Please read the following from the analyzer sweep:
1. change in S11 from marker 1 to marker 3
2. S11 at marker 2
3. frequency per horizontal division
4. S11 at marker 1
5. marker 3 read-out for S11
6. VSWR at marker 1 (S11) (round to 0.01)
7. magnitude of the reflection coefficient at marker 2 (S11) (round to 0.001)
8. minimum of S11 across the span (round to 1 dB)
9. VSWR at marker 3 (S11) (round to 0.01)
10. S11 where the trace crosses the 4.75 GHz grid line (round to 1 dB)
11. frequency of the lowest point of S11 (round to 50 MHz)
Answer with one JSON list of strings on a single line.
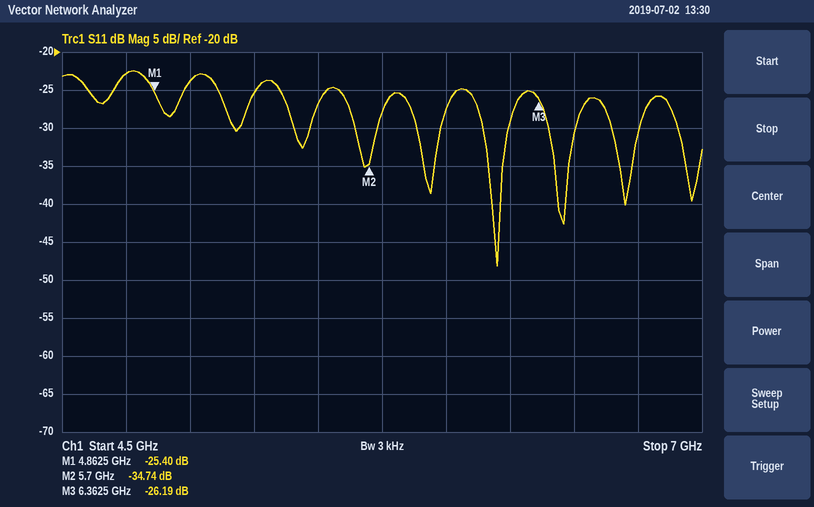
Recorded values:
["-0.79 dB", "-34.74 dB", "250 MHz", "-25.40 dB", "-26.19 dB", "1.11", "0.018", "-48 dB", "1.10", "-23 dB", "6.20 GHz"]
